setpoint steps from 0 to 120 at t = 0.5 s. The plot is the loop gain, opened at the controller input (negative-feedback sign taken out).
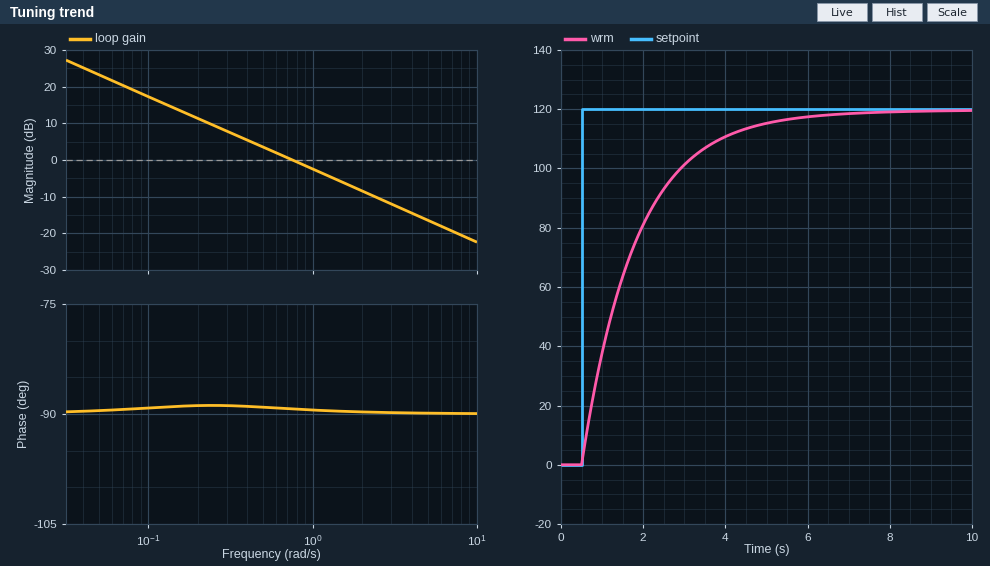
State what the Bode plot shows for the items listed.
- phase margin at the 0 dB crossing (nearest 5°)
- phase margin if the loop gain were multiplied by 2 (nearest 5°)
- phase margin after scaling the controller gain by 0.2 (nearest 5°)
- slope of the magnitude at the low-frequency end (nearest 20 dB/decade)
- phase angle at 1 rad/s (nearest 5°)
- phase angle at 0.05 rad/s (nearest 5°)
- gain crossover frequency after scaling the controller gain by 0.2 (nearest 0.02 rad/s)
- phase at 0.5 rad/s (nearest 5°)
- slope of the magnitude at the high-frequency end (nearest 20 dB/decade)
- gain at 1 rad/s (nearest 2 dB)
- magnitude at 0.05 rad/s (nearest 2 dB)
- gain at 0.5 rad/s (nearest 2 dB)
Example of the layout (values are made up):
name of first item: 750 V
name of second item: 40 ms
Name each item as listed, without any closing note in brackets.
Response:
phase margin at the 0 dB crossing: 90°
phase margin if the loop gain were multiplied by 2: 90°
phase margin after scaling the controller gain by 0.2: 90°
slope of the magnitude at the low-frequency end: -20 dB/decade
phase angle at 1 rad/s: -90°
phase angle at 0.05 rad/s: -90°
gain crossover frequency after scaling the controller gain by 0.2: 0.14 rad/s
phase at 0.5 rad/s: -90°
slope of the magnitude at the high-frequency end: -20 dB/decade
gain at 1 rad/s: -2 dB
magnitude at 0.05 rad/s: 24 dB
gain at 0.5 rad/s: 4 dB
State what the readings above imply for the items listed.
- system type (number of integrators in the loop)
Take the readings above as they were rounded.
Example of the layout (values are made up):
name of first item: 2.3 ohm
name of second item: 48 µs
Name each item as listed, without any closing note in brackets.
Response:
system type: 1
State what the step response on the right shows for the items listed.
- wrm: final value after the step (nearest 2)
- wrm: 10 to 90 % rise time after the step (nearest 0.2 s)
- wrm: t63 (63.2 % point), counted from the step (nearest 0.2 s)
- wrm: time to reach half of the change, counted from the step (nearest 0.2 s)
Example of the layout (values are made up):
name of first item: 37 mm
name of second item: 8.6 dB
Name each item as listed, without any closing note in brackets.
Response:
wrm: final value after the step: 120
wrm: 10 to 90 % rise time after the step: 3.0 s
wrm: t63 (63.2 % point), counted from the step: 1.4 s
wrm: time to reach half of the change, counted from the step: 1.0 s
